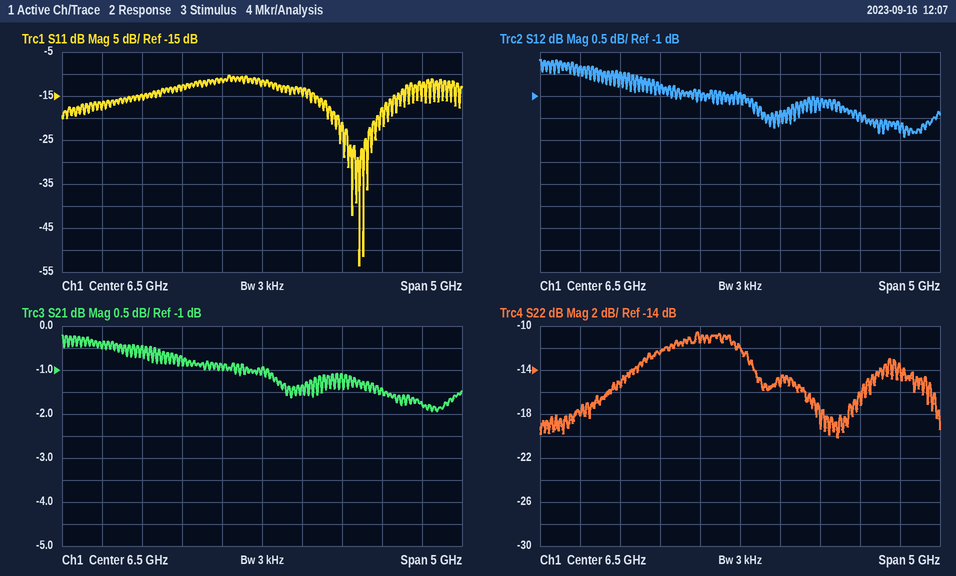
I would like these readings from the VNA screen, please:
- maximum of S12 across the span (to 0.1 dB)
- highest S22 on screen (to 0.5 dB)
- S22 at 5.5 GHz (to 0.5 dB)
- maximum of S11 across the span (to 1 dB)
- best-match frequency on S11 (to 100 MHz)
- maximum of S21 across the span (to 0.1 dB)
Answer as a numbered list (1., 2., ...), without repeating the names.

1. -0.2 dB
2. -10.5 dB
3. -12.5 dB
4. -10 dB
5. 7.7 GHz
6. -0.2 dB
